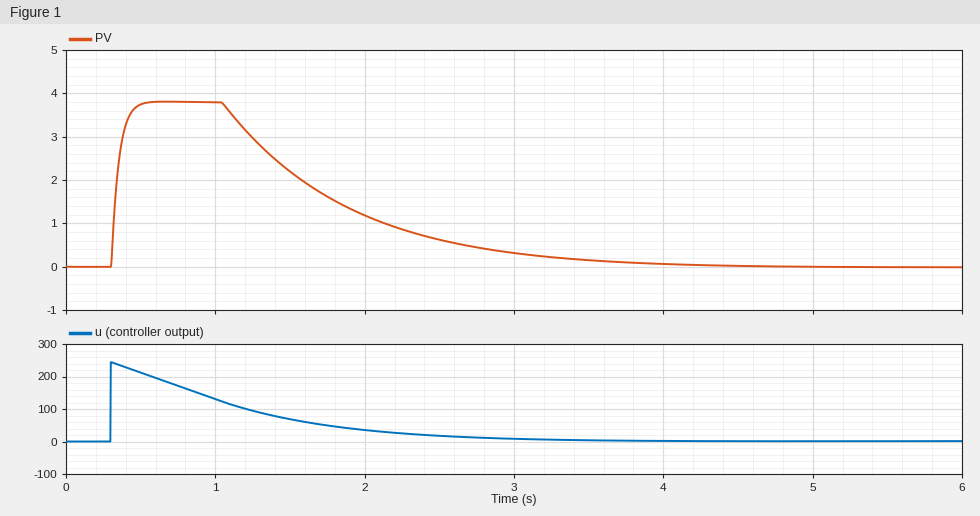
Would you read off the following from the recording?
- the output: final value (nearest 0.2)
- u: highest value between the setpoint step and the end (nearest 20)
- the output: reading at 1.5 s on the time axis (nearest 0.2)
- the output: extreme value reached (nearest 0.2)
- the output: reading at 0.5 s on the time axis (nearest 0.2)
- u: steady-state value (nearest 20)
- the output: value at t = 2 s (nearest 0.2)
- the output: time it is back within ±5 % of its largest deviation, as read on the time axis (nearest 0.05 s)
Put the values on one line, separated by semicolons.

0.0; 240; 2.2; 3.8; 3.8; 0; 1.2; 3.35 s
